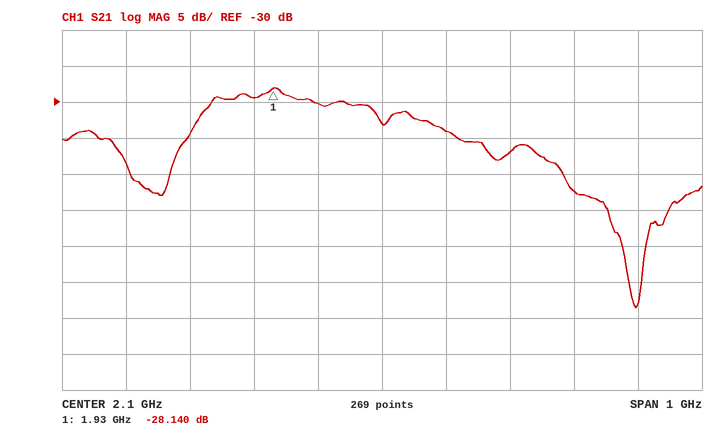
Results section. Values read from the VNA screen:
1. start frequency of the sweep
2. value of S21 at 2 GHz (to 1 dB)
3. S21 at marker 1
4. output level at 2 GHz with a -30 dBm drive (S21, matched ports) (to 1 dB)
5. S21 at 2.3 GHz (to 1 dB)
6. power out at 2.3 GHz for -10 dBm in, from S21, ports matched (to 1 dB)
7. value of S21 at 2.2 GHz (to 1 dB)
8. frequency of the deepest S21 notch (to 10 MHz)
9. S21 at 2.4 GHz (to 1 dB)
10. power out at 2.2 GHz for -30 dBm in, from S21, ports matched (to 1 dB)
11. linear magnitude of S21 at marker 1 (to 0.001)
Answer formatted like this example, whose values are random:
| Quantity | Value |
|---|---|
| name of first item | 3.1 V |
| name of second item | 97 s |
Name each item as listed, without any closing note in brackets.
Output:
| Quantity | Value |
|---|---|
| start frequency of the sweep | 1.6 GHz |
| value of S21 at 2 GHz | -30 dB |
| S21 at marker 1 | -28.140 dB |
| output level at 2 GHz with a -30 dBm drive (S21, matched ports) | -60 dBm |
| S21 at 2.3 GHz | -37 dB |
| power out at 2.3 GHz for -10 dBm in, from S21, ports matched | -47 dBm |
| value of S21 at 2.2 GHz | -34 dB |
| frequency of the deepest S21 notch | 2.50 GHz |
| S21 at 2.4 GHz | -42 dB |
| power out at 2.2 GHz for -30 dBm in, from S21, ports matched | -64 dBm |
| linear magnitude of S21 at marker 1 | 0.039 |
